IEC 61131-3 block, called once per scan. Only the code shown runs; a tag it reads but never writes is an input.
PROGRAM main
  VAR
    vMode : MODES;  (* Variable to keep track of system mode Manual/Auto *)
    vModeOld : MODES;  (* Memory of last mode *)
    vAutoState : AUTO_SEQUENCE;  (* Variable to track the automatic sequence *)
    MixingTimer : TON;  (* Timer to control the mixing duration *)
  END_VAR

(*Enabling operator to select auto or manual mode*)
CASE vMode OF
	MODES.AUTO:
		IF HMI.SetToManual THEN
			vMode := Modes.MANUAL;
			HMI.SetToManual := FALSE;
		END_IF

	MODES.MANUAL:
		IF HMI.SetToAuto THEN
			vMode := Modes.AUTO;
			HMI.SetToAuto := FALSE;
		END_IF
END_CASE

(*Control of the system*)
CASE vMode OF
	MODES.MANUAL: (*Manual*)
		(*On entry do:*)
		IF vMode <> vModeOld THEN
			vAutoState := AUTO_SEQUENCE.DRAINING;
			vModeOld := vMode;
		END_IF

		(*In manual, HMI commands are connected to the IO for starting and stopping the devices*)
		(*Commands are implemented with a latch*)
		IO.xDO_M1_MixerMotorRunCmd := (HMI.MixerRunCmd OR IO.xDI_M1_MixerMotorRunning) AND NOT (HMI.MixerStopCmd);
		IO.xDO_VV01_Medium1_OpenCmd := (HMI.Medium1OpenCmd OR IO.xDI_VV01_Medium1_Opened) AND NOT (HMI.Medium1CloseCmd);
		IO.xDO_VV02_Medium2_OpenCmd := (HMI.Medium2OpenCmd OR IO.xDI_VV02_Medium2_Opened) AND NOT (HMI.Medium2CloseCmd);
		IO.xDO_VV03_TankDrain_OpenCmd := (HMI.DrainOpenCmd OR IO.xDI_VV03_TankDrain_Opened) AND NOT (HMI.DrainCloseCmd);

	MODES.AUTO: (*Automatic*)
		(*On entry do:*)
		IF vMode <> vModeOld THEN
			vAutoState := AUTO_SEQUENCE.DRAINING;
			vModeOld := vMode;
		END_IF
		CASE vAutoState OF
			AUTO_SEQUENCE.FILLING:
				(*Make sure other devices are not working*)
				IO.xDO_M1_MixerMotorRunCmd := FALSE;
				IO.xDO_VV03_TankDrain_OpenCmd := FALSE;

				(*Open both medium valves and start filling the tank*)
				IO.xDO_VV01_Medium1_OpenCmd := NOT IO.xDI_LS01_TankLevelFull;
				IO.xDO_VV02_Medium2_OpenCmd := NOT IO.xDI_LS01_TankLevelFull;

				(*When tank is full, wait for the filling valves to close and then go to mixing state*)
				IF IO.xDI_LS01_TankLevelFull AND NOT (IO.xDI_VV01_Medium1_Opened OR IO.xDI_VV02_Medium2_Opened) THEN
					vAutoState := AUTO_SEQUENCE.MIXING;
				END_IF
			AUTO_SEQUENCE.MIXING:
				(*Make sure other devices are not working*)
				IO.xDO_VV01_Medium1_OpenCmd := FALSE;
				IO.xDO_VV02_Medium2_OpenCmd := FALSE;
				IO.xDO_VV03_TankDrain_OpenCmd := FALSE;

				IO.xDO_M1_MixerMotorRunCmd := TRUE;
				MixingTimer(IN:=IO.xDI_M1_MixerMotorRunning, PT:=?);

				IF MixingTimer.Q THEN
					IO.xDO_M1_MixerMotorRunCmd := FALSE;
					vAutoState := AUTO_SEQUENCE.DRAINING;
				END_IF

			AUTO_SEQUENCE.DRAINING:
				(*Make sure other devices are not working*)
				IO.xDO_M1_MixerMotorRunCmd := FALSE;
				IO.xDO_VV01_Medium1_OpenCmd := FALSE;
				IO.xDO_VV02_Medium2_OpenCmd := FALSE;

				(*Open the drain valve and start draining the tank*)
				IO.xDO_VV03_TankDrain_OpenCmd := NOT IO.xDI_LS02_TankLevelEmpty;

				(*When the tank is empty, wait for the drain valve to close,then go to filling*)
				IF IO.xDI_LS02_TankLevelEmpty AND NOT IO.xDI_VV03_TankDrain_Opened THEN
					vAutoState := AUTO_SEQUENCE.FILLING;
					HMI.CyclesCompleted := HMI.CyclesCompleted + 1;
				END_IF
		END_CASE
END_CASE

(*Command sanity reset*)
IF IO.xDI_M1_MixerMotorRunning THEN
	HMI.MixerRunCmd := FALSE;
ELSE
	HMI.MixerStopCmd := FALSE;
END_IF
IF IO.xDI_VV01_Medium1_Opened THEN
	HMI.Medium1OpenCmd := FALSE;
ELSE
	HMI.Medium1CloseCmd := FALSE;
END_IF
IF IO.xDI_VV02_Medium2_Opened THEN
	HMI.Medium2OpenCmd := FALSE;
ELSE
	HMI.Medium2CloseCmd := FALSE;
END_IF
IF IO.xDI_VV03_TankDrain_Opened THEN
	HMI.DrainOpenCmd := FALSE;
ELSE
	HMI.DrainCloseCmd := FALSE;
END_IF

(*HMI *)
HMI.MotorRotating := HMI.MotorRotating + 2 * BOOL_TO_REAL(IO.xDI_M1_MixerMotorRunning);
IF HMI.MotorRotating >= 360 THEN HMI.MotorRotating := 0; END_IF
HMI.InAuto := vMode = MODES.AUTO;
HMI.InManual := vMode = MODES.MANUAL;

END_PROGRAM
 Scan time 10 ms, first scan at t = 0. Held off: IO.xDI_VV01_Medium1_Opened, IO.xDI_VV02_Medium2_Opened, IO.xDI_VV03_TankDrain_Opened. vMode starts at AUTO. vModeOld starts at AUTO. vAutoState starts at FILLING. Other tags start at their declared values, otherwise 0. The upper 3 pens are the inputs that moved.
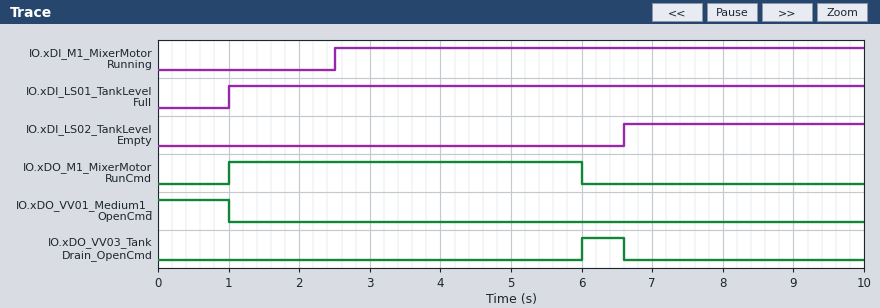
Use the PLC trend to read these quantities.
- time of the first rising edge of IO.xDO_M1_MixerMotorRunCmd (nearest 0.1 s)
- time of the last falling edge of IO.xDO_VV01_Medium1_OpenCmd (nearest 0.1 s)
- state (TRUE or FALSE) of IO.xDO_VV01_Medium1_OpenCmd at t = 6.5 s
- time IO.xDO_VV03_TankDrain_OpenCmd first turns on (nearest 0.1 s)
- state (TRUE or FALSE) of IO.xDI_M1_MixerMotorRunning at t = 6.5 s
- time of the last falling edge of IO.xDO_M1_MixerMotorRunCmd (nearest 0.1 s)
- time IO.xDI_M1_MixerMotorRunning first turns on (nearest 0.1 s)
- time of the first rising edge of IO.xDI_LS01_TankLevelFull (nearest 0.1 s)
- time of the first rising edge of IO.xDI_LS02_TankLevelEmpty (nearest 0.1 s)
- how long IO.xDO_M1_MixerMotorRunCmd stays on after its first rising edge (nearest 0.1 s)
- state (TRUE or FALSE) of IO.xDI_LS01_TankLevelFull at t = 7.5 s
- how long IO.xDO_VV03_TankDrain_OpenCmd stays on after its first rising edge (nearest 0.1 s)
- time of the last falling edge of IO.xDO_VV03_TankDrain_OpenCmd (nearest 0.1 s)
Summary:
1.0 s
1.0 s
FALSE
6.0 s
TRUE
6.0 s
2.5 s
1.0 s
6.6 s
5.0 s
TRUE
0.6 s
6.6 s
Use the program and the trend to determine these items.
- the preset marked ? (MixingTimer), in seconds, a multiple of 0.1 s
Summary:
3.5 s
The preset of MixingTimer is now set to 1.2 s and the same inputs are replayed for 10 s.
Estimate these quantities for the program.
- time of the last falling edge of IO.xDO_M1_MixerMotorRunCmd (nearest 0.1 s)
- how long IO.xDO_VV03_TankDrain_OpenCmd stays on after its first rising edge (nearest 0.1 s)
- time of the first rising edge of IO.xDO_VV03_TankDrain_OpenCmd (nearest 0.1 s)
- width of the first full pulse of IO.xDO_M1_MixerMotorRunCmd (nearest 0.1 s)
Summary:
3.7 s
2.9 s
3.7 s
2.7 s
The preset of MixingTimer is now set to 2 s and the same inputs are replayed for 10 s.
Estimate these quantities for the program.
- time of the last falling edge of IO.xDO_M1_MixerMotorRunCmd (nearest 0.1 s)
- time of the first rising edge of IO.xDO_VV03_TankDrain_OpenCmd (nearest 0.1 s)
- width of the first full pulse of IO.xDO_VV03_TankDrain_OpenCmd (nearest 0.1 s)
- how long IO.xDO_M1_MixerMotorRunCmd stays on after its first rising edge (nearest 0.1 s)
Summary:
4.5 s
4.5 s
2.1 s
3.5 s
